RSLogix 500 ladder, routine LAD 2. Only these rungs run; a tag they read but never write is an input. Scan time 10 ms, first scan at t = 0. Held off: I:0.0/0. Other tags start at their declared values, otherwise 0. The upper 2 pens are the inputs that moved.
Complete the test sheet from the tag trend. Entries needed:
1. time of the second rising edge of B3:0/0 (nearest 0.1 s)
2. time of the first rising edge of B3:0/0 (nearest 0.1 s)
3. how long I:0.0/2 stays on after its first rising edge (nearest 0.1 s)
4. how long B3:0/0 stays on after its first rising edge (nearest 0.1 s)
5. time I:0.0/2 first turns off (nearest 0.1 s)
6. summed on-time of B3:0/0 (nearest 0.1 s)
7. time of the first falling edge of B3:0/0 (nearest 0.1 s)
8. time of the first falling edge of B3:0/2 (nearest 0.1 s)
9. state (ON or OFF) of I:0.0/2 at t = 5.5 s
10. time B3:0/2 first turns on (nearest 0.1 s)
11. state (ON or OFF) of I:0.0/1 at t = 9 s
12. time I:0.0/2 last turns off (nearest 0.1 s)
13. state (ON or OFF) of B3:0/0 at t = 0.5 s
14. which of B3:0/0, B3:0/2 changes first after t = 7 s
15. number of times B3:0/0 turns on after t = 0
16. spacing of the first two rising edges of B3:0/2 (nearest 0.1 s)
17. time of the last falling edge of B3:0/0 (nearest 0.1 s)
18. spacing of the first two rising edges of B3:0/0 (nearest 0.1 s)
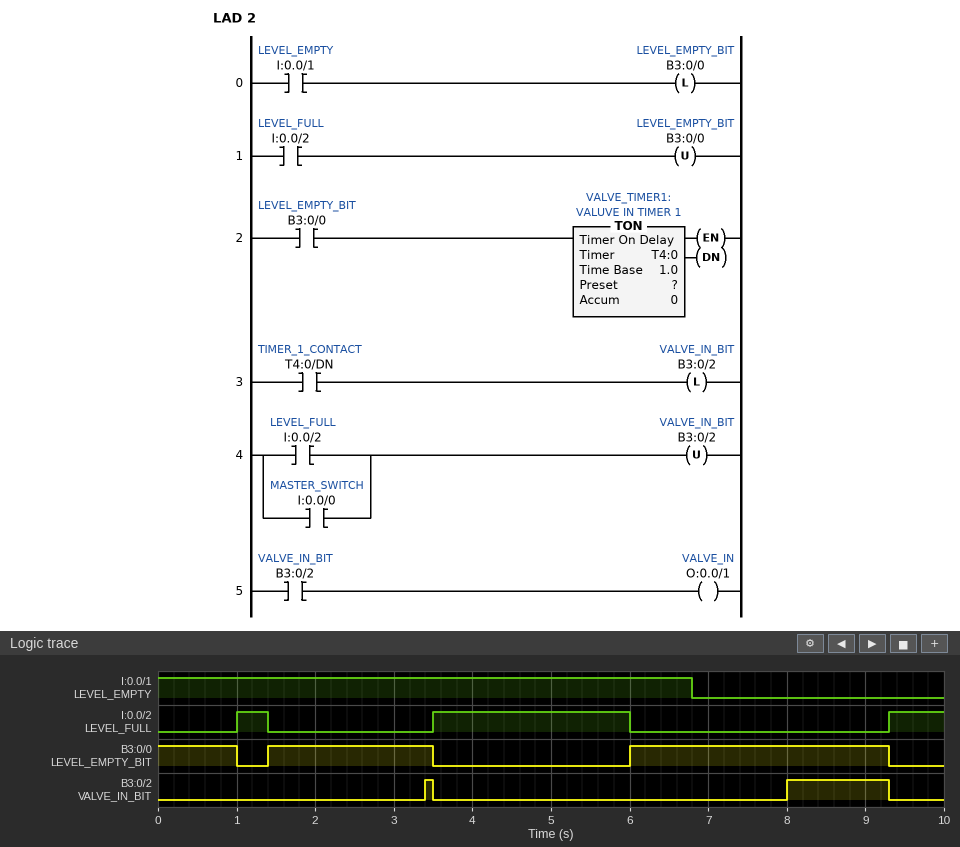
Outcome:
6.0 s
1.4 s
0.4 s
2.1 s
1.4 s
6.4 s
1.0 s
3.5 s
ON
3.4 s
OFF
6.0 s
ON
B3:0/2
2
4.6 s
9.3 s
4.6 s
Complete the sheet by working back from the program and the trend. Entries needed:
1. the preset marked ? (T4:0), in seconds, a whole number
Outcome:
2 s
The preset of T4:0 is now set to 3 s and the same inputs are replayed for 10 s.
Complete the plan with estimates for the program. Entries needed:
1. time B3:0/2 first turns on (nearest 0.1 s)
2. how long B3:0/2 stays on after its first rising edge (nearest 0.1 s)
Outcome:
9.0 s
0.3 s
